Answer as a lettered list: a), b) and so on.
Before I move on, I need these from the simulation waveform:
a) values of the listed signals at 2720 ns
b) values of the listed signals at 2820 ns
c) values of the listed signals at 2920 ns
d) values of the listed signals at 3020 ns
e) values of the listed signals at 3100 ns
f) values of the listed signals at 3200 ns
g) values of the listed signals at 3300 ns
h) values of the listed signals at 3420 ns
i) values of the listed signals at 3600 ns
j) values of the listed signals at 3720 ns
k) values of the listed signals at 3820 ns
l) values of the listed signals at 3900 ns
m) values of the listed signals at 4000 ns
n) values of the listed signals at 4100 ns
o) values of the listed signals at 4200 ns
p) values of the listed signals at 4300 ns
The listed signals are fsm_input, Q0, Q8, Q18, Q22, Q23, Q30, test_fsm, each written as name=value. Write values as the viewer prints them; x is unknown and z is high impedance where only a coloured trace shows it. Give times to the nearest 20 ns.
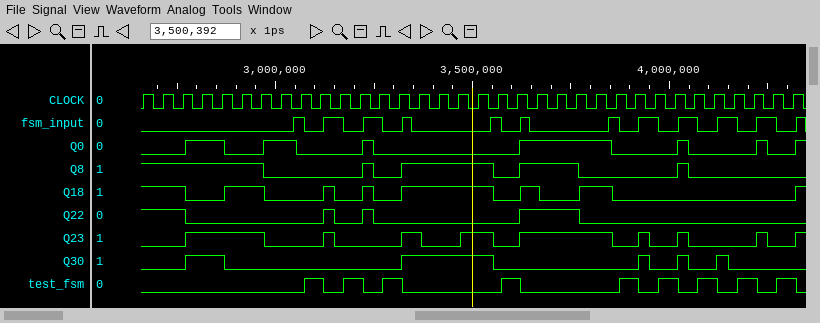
a) fsm_input=0, Q0=0, Q8=1, Q18=1, Q22=1, Q23=0, Q30=0, test_fsm=0
b) fsm_input=0, Q0=1, Q8=1, Q18=0, Q22=0, Q23=1, Q30=1, test_fsm=0
c) fsm_input=0, Q0=0, Q8=1, Q18=1, Q22=0, Q23=1, Q30=0, test_fsm=0
d) fsm_input=0, Q0=1, Q8=0, Q18=0, Q22=0, Q23=0, Q30=0, test_fsm=0
e) fsm_input=0, Q0=0, Q8=0, Q18=0, Q22=0, Q23=0, Q30=0, test_fsm=1
f) fsm_input=0, Q0=0, Q8=0, Q18=0, Q22=0, Q23=0, Q30=0, test_fsm=1
g) fsm_input=0, Q0=0, Q8=0, Q18=0, Q22=0, Q23=0, Q30=0, test_fsm=1
h) fsm_input=0, Q0=0, Q8=1, Q18=1, Q22=0, Q23=0, Q30=1, test_fsm=0
i) fsm_input=0, Q0=0, Q8=0, Q18=0, Q22=0, Q23=0, Q30=0, test_fsm=1
j) fsm_input=0, Q0=1, Q8=1, Q18=0, Q22=1, Q23=1, Q30=0, test_fsm=0
k) fsm_input=0, Q0=1, Q8=0, Q18=1, Q22=0, Q23=1, Q30=0, test_fsm=0
l) fsm_input=0, Q0=0, Q8=0, Q18=0, Q22=0, Q23=0, Q30=0, test_fsm=1
m) fsm_input=0, Q0=0, Q8=0, Q18=0, Q22=0, Q23=0, Q30=0, test_fsm=1
n) fsm_input=0, Q0=0, Q8=0, Q18=0, Q22=0, Q23=0, Q30=0, test_fsm=1
o) fsm_input=0, Q0=0, Q8=0, Q18=0, Q22=0, Q23=0, Q30=0, test_fsm=1
p) fsm_input=0, Q0=0, Q8=0, Q18=0, Q22=0, Q23=0, Q30=0, test_fsm=1
